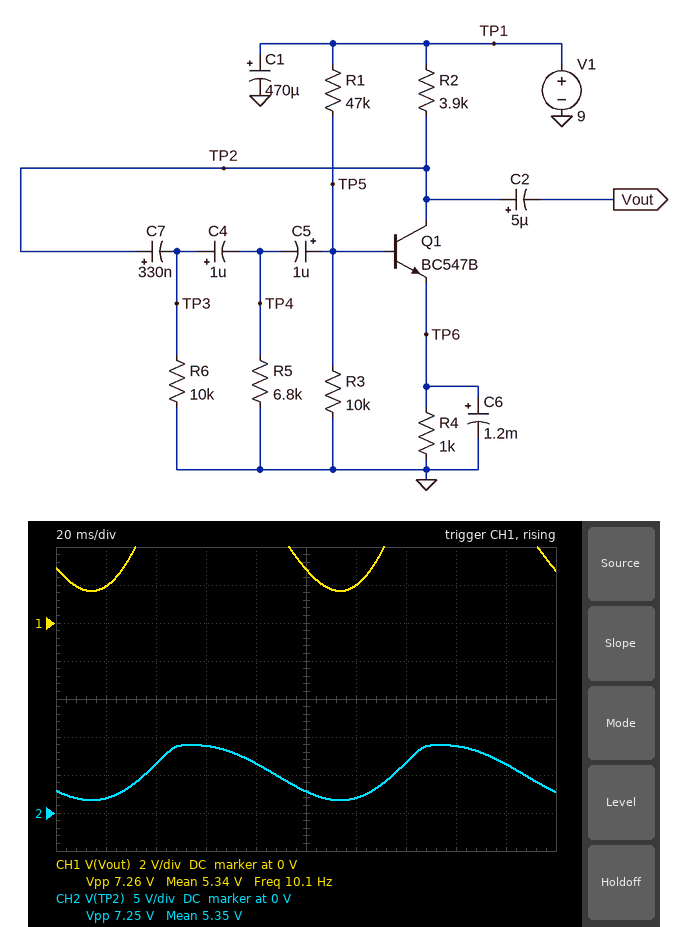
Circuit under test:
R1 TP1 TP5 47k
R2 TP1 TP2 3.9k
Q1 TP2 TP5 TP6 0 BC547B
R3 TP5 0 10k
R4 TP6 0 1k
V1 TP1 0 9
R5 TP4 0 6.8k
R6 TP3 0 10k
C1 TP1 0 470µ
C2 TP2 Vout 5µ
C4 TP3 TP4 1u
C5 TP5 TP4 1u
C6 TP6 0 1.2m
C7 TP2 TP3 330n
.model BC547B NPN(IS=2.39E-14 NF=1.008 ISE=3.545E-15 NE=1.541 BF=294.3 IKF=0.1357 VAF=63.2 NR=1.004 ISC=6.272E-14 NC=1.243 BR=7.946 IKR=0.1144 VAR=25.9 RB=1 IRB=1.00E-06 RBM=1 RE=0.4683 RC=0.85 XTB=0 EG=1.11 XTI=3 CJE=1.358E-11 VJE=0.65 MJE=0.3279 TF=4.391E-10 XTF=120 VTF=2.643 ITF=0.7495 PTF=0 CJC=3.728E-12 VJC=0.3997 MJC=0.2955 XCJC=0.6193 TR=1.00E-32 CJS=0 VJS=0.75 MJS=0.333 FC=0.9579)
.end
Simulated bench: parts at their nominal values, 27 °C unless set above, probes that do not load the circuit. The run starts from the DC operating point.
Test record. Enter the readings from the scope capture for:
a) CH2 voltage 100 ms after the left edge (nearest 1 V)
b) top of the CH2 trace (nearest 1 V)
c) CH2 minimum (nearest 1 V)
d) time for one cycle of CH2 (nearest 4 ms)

3 V
9 V
2 V
100 ms
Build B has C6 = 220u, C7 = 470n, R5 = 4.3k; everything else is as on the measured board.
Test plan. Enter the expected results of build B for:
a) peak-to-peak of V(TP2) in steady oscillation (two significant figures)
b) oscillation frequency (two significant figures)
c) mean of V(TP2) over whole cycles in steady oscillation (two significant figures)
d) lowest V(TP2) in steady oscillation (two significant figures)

7.9 V
13 Hz
5.4 V
980 mV
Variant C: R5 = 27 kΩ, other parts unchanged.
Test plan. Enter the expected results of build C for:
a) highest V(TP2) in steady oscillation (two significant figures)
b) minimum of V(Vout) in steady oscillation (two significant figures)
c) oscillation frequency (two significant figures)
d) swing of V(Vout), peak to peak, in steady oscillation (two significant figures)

8.9 V
2.0 V
7.3 Hz
6.9 V
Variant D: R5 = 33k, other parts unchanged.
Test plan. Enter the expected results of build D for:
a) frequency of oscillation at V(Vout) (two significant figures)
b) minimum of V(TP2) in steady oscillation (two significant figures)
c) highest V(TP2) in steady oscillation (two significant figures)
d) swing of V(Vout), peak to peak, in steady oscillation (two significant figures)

7.0 Hz
2.1 V
8.9 V
6.8 V
